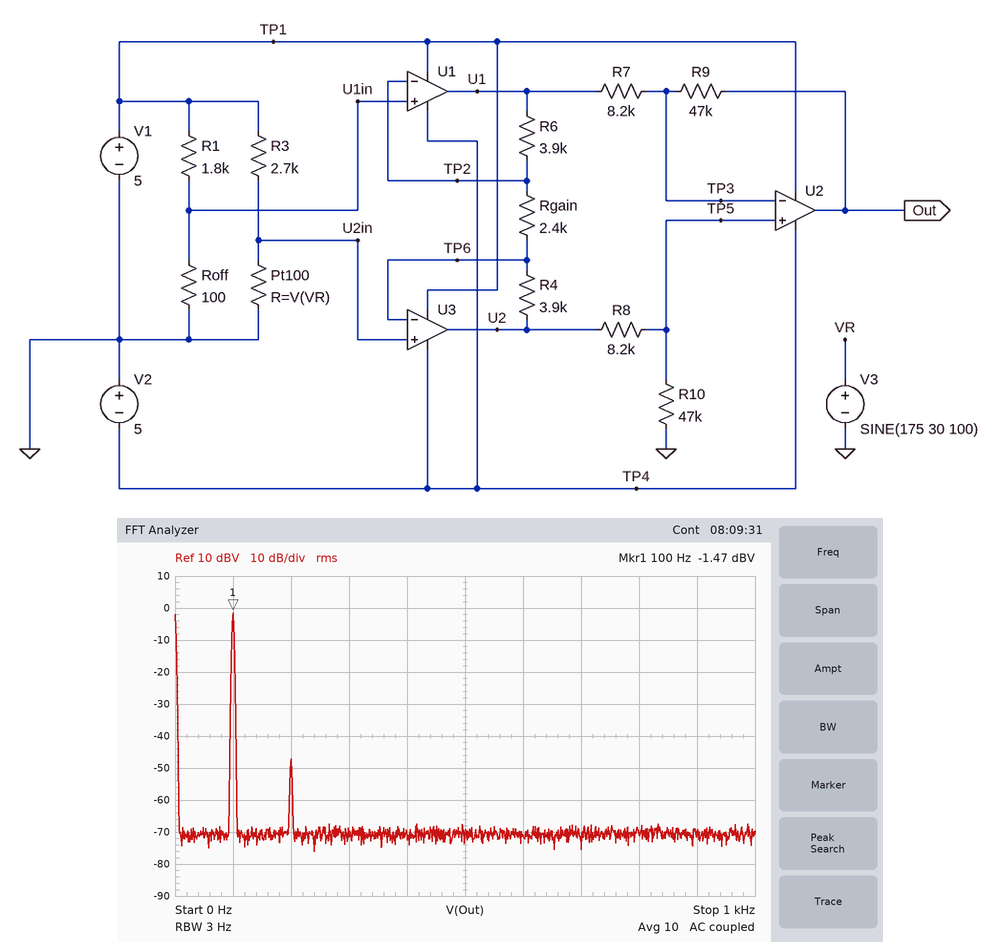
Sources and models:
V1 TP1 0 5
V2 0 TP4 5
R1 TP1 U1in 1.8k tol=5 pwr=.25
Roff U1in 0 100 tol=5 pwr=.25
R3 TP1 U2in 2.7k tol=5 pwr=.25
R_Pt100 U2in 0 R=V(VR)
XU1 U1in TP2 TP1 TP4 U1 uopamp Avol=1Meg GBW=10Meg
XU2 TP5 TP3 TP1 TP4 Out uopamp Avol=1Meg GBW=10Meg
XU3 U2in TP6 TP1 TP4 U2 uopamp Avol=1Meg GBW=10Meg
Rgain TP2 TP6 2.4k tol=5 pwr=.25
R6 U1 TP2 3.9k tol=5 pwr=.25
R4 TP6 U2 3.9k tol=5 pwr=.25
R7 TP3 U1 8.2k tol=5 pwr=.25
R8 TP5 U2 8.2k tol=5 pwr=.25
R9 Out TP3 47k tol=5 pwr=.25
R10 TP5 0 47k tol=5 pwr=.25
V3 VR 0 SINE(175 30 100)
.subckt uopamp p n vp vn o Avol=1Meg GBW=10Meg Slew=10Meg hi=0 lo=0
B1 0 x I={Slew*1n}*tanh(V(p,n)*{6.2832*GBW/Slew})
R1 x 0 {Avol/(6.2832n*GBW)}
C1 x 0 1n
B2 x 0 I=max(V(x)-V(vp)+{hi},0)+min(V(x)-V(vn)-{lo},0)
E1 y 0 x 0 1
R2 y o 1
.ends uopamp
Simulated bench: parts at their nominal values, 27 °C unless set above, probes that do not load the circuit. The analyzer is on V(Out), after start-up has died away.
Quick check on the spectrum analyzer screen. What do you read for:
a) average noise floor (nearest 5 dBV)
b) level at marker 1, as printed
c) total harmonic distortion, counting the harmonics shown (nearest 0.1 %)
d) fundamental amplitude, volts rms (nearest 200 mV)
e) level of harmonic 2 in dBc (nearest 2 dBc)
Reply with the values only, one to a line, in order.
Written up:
-70 dBV
-1.47 dBV
0.5 %
800 mV
-46 dBc
